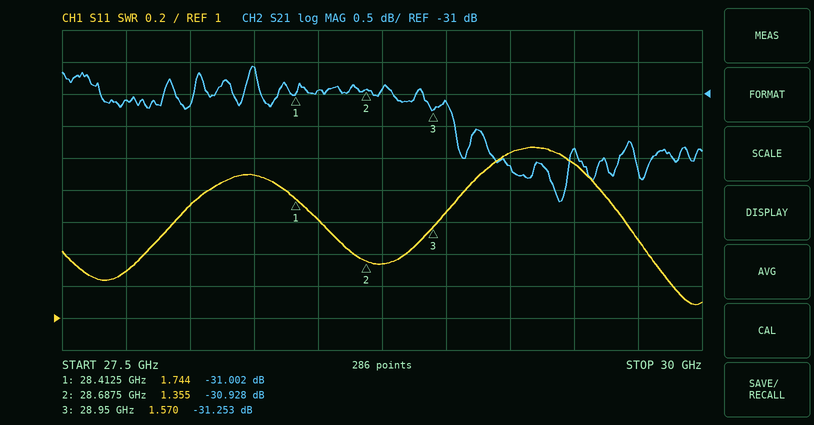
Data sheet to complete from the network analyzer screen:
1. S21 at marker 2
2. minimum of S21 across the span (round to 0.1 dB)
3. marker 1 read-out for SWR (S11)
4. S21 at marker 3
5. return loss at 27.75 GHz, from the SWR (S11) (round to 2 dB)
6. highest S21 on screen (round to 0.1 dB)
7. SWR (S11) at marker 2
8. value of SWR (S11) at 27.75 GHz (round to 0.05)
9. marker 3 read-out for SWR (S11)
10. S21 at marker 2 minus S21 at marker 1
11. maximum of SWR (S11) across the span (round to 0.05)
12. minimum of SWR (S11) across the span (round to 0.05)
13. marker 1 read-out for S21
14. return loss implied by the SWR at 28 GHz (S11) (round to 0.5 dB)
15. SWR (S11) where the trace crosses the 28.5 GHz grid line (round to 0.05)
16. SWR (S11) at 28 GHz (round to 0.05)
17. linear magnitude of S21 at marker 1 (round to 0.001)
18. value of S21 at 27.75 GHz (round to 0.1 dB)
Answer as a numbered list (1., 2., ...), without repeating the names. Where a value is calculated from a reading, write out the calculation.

1. -30.928 dB
2. -32.7 dB
3. 1.744
4. -31.253 dB
5. −20 log10((1.3 − 1)/(1.3 + 1)) ≈ 18 dB
6. -30.6 dB
7. 1.355
8. 1.30
9. 1.570
10. -30.928 − (-31.002) = 0.074 dB
11. 2.05
12. 1.10
13. -31.002 dB
14. −20 log10((1.7 − 1)/(1.7 + 1)) ≈ 11.7 dB, so 11.5 dB to the nearest 0.5 dB
15. 1.60
16. 1.70
17. 10^(-31.002/20) ≈ 0.028
18. -31.1 dB
